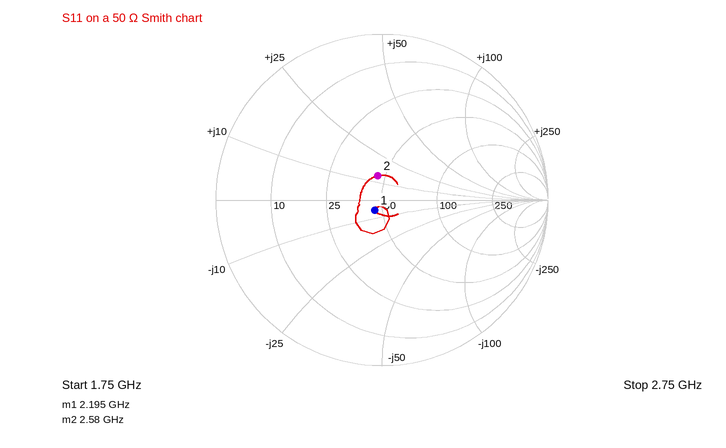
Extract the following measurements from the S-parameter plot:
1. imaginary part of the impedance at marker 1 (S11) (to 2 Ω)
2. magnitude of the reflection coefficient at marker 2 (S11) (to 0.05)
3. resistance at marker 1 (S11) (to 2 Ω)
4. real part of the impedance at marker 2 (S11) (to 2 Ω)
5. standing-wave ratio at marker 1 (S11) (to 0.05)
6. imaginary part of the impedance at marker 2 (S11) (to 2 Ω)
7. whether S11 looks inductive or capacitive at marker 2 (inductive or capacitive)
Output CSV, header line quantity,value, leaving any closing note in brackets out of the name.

quantity,value
imaginary part of the impedance at marker 1 (S11),-6 Ω
magnitude of the reflection coefficient at marker 2 (S11),0.15
resistance at marker 1 (S11),46 Ω
real part of the impedance at marker 2 (S11),46 Ω
standing-wave ratio at marker 1 (S11),1.15
imaginary part of the impedance at marker 2 (S11),+14 Ω
whether S11 looks inductive or capacitive at marker 2,inductive
